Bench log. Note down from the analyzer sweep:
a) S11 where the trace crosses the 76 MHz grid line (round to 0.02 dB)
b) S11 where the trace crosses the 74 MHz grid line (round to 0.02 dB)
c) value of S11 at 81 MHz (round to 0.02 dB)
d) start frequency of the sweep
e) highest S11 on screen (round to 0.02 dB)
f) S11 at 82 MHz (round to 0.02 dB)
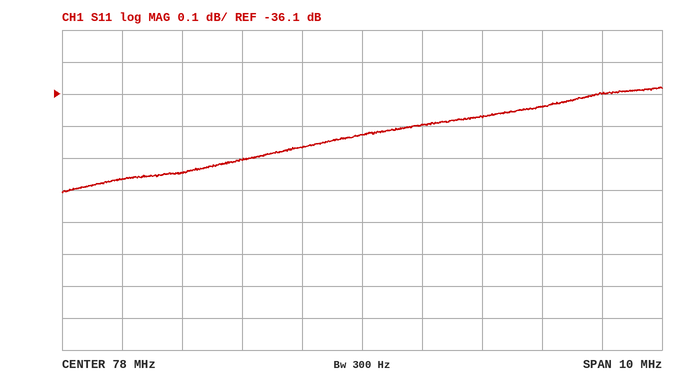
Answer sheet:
-36.30 dB
-36.36 dB
-36.14 dB
73 MHz
-36.08 dB
-36.10 dB
